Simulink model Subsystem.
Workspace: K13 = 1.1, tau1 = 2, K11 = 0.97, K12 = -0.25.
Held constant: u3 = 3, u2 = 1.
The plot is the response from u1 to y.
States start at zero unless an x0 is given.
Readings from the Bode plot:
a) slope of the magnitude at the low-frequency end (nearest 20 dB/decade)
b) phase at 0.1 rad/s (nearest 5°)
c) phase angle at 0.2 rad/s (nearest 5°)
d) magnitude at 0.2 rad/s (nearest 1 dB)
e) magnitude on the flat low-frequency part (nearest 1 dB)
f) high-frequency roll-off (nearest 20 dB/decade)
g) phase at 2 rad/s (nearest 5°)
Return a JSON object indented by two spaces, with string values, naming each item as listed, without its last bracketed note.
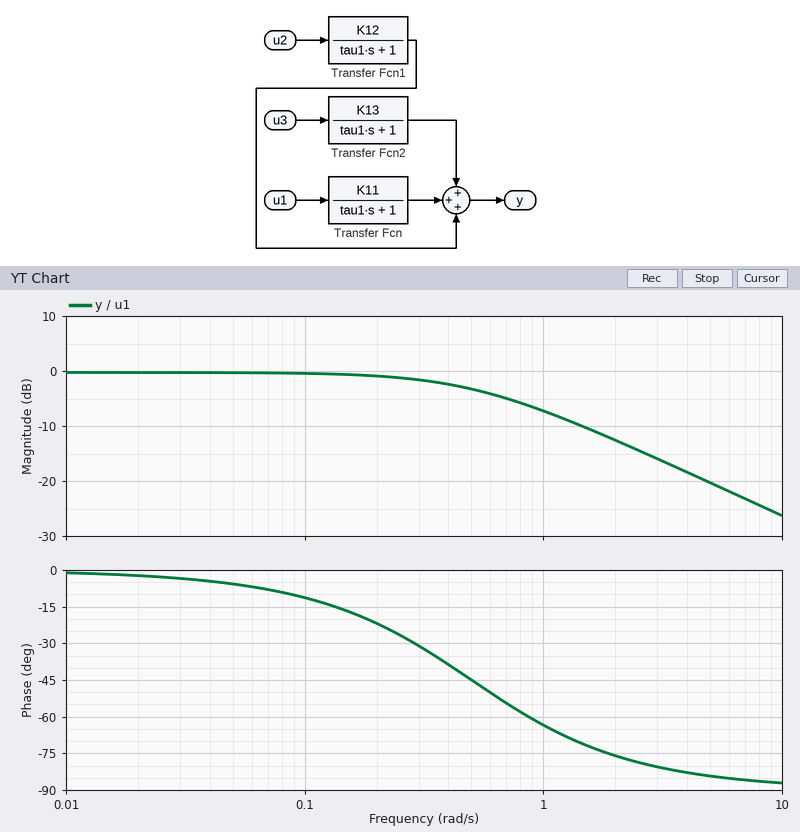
{
  "slope of the magnitude at the low-frequency end": "0 dB/decade",
  "phase at 0.1 rad/s": "-10°",
  "phase angle at 0.2 rad/s": "-20°",
  "magnitude at 0.2 rad/s": "-1 dB",
  "magnitude on the flat low-frequency part": "0 dB",
  "high-frequency roll-off": "-20 dB/decade",
  "phase at 2 rad/s": "-75°"
}
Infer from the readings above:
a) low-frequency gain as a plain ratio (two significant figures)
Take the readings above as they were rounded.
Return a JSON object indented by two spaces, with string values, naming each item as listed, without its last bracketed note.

{
  "low-frequency gain as a plain ratio": "1.0"
}
